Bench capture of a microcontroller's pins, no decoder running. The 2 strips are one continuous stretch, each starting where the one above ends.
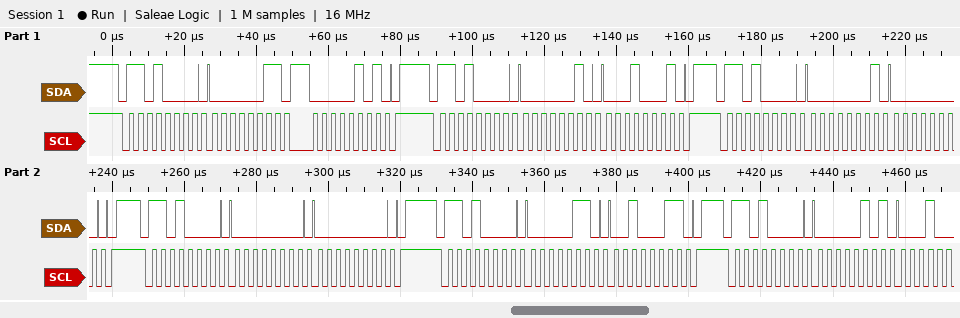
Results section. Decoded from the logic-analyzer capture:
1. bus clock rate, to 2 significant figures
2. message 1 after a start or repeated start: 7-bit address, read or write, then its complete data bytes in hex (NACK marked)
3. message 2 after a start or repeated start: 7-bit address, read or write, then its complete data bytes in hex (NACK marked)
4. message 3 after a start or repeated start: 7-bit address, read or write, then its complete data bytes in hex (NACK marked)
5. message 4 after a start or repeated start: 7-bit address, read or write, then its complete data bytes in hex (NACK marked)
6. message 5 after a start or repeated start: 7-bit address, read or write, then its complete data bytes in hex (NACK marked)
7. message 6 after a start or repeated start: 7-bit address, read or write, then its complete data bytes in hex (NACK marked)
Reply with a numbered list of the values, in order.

1. 400 kHz
2. 0x68 write: 03 05
3. 0x68 write: 02 11
4. 0x68 write: 01 00
5. 0x68 write: 00 00
6. 0x68 write: 06 23
7. 0x68 write: 05
